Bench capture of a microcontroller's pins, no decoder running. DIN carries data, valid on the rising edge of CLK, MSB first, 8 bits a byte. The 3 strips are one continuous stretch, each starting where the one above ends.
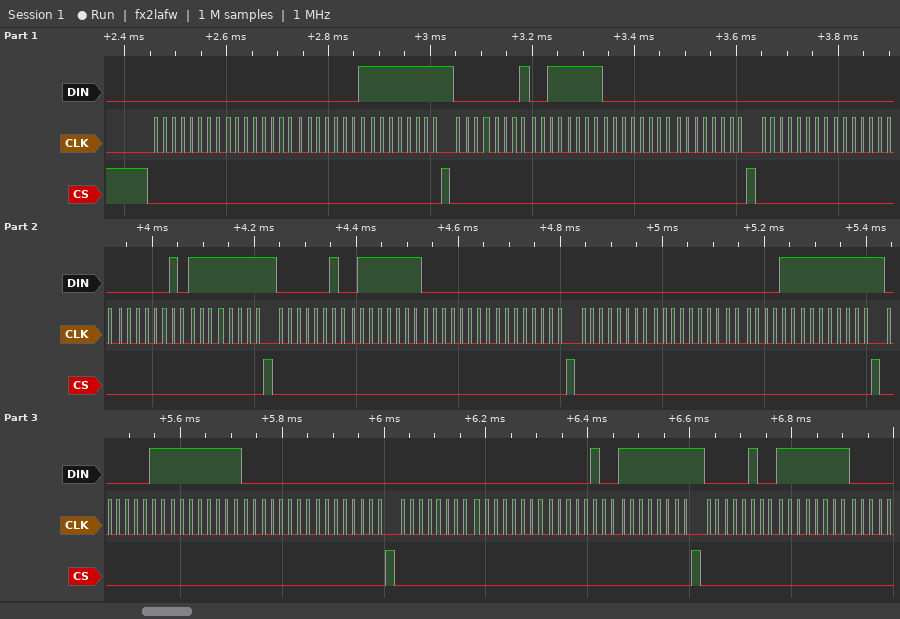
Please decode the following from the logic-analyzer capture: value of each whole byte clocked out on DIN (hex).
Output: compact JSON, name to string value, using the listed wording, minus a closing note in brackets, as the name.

{"value of each whole byte clocked out on DIN": "00 00 01 FF 01 3F 00 00 00 00 02 FF 02 7F 00 00 00 00 03 FF 03 FF 00 00 00 00 04 FF 04 FF"}
